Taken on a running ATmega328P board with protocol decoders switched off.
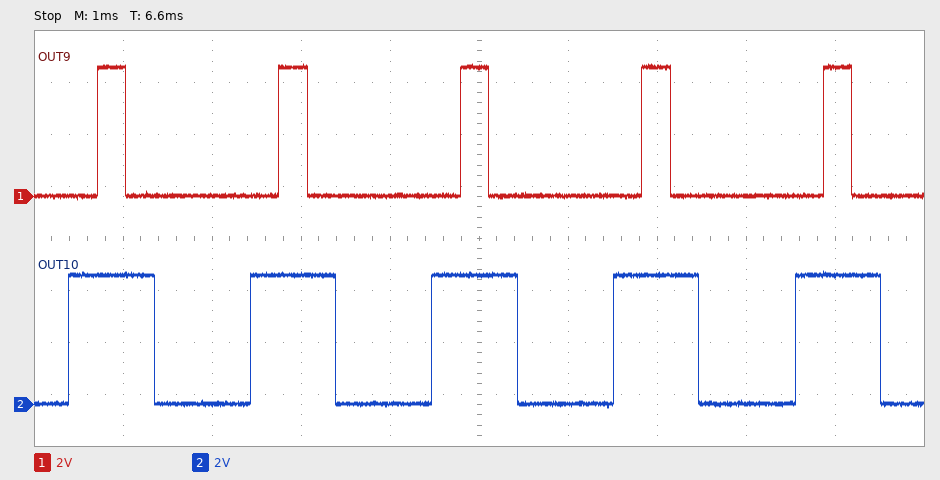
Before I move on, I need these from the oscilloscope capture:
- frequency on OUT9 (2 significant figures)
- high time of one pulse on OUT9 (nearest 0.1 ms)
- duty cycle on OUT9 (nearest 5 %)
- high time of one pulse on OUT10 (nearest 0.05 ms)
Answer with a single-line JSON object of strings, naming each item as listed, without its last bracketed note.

{"frequency on OUT9": "490 Hz", "high time of one pulse on OUT9": "0.3 ms", "duty cycle on OUT9": "15 %", "high time of one pulse on OUT10": "0.95 ms"}
